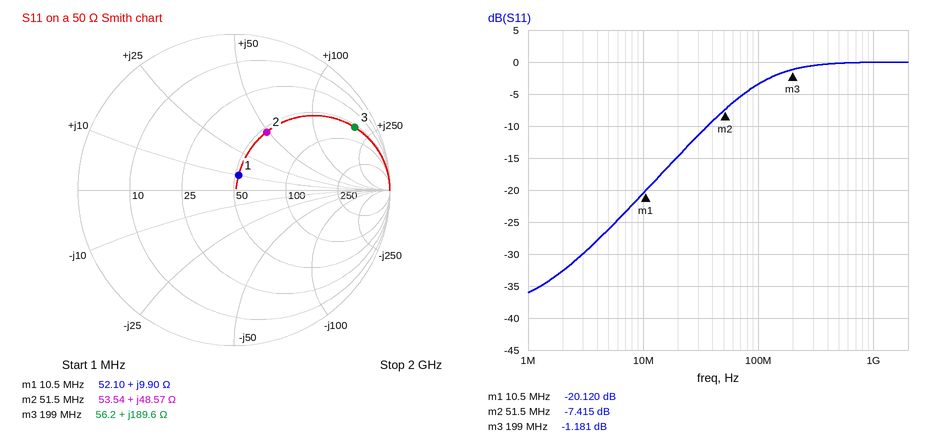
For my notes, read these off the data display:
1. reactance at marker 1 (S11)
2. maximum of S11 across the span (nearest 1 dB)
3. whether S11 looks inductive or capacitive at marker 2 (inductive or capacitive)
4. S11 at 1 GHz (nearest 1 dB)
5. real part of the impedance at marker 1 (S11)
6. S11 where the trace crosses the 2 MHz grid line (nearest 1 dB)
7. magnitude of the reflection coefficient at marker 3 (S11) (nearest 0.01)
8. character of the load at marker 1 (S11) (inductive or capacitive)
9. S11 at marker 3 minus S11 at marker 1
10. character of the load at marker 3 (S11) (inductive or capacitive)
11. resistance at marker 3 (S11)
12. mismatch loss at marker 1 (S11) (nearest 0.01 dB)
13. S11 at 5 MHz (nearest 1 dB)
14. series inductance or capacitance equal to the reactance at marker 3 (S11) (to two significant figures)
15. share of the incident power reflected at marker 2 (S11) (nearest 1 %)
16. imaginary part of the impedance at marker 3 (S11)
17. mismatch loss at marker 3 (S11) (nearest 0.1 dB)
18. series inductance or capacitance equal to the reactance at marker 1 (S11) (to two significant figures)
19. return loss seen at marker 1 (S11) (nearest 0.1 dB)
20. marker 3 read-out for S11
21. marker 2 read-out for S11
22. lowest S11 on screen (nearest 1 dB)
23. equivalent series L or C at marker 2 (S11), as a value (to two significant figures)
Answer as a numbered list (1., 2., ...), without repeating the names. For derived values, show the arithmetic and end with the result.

1. +9.90 Ω
2. 0 dB
3. inductive
4. 0 dB
5. 52.10 Ω
6. -33 dB
7. 0.87
8. inductive
9. -1.181 − (-20.12) = 18.939 dB
10. inductive
11. 56.2 Ω
12. −10 log10(1 − 10^(-20.12/10)) ≈ 0.04 dB
13. -26 dB
14. L = 189.6 Ω/(2π × 199 MHz) ≈ 152 nH, so 150 nH to two significant figures
15. 10^(-7.415/10) ≈ 18 %
16. +189.6 Ω
17. −10 log10(1 − 10^(-1.181/10)) ≈ 6.2 dB
18. L = 9.9 Ω/(2π × 10.5 MHz) ≈ 150 nH
19. 20.1 dB
20. -1.181 dB
21. -7.415 dB
22. -36 dB
23. L = 48.57 Ω/(2π × 51.5 MHz) ≈ 150 nH
